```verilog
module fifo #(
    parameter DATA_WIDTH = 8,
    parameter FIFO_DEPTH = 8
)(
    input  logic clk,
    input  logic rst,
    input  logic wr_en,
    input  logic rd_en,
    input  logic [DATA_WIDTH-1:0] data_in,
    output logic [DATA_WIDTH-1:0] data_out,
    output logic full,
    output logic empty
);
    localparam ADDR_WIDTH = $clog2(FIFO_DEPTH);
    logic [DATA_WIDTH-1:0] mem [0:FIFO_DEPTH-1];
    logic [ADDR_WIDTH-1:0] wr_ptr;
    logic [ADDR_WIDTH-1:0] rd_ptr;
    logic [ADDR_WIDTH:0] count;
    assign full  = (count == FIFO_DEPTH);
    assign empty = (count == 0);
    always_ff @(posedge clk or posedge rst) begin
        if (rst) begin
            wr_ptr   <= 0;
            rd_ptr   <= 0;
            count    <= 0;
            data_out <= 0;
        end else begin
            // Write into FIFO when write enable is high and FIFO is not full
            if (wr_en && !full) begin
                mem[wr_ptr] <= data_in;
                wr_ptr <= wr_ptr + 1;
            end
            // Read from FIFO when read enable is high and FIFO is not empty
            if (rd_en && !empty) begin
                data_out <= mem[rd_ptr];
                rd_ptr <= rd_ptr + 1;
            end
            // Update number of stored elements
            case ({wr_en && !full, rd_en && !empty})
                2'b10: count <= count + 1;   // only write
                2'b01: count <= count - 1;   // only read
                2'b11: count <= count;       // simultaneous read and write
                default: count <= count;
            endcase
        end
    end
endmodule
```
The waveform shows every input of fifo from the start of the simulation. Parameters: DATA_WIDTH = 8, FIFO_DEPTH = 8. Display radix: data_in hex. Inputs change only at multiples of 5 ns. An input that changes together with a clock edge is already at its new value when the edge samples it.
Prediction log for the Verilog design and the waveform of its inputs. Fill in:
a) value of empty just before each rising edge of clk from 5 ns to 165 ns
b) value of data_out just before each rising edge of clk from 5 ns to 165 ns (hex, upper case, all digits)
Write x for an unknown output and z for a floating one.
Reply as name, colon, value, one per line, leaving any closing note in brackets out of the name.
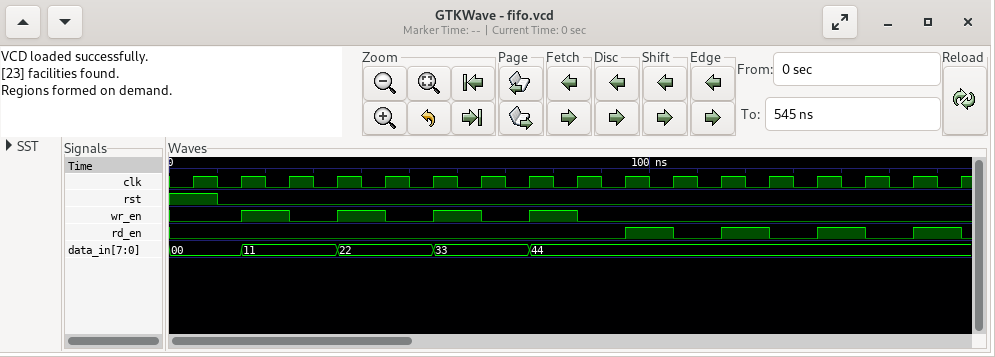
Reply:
value of empty just before each rising edge of clk from 5 ns to 165 ns: 1 1 0 0 0 0 0 0 0 0 0 0 0 0 0 0 1
value of data_out just before each rising edge of clk from 5 ns to 165 ns: 00, 00, 00, 00, 00, 00, 00, 00, 00, 00, 11, 11, 22, 22, 33, 33, 44
